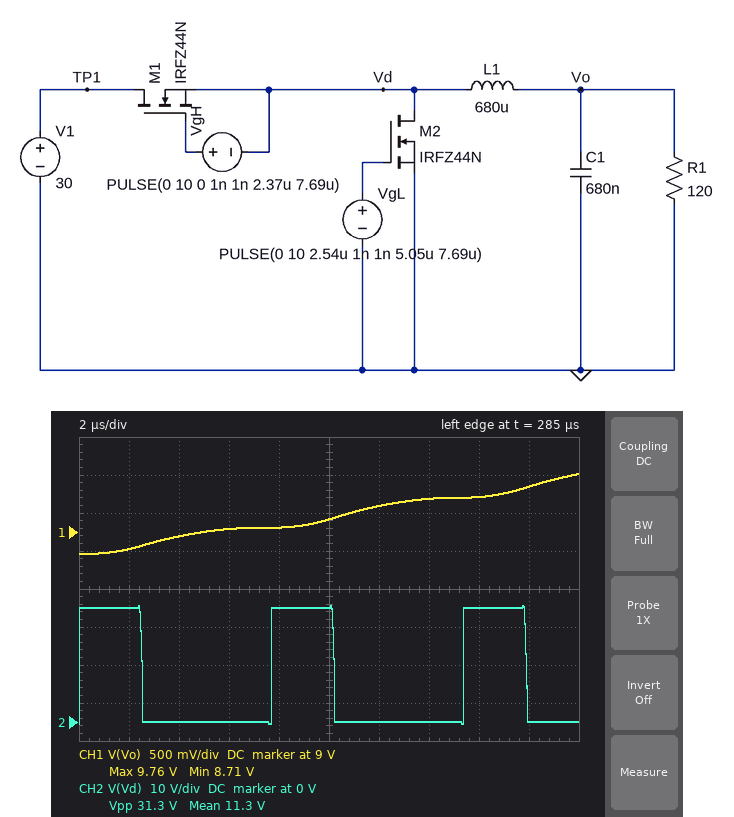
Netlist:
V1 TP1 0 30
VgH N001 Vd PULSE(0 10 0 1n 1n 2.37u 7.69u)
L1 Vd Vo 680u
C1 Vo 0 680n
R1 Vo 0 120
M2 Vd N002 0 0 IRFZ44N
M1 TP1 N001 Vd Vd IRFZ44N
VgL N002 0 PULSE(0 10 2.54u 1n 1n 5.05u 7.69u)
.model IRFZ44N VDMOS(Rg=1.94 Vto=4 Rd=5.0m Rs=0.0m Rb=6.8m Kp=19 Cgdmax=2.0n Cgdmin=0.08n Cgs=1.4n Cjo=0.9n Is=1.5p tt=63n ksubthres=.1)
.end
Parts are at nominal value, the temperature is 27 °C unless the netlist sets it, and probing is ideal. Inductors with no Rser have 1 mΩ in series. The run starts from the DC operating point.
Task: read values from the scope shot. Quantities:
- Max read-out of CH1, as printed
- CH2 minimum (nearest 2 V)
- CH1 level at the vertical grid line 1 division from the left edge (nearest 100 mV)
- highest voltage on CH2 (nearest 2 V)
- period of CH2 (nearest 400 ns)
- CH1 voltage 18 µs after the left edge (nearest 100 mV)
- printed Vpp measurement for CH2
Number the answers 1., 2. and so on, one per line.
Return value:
1. 9.76 V
2. 0 V
3. 8.8 V
4. 30 V
5. 7.6 µs
6. 9.6 V
7. 31.3 V
